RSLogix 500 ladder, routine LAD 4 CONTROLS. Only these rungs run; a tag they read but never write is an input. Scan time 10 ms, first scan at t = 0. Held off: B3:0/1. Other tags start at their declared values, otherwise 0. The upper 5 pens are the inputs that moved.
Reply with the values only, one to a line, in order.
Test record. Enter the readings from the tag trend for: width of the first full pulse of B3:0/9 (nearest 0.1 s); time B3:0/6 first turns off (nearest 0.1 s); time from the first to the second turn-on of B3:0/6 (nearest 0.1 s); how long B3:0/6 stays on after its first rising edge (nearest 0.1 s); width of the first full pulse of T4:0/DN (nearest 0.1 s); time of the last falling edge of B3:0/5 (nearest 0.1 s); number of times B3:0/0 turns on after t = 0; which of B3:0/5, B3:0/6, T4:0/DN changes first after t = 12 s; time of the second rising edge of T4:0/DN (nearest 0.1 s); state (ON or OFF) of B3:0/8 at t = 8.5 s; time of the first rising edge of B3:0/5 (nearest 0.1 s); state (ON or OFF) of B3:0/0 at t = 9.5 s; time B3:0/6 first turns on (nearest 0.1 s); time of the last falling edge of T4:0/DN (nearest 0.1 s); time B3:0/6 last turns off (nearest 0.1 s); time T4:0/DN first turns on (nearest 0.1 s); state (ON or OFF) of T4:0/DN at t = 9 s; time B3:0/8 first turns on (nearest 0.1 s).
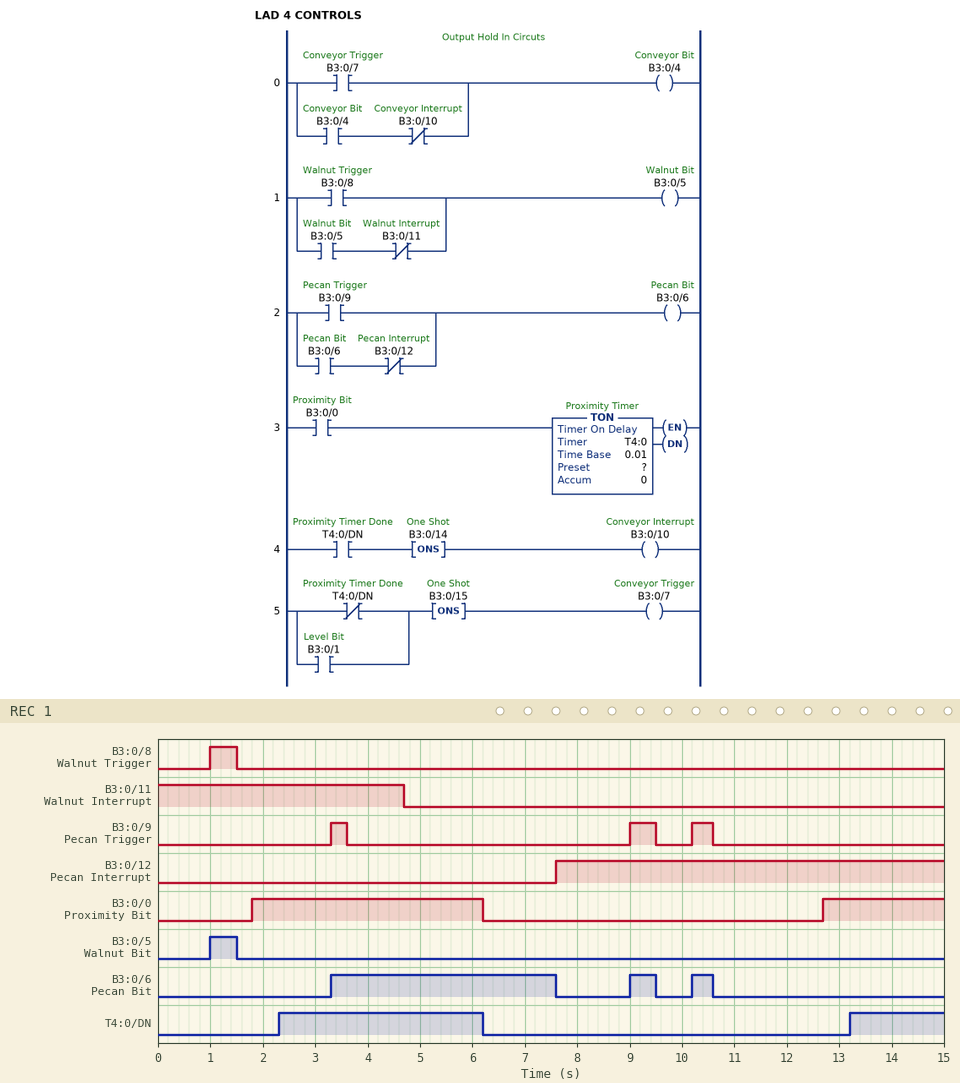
0.3 s
7.6 s
5.7 s
4.3 s
3.9 s
1.5 s
2
T4:0/DN
13.2 s
OFF
1.0 s
OFF
3.3 s
6.2 s
10.6 s
2.3 s
OFF
1.0 s
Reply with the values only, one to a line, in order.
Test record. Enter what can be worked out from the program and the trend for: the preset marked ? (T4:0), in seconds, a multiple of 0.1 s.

0.5 s
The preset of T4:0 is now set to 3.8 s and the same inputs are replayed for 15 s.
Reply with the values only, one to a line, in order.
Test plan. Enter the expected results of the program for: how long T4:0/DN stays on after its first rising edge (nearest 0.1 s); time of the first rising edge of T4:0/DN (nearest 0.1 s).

0.6 s
5.6 s
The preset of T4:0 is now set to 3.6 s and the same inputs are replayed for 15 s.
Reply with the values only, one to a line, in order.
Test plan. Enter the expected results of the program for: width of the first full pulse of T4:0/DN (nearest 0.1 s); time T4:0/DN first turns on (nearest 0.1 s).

0.8 s
5.4 s
